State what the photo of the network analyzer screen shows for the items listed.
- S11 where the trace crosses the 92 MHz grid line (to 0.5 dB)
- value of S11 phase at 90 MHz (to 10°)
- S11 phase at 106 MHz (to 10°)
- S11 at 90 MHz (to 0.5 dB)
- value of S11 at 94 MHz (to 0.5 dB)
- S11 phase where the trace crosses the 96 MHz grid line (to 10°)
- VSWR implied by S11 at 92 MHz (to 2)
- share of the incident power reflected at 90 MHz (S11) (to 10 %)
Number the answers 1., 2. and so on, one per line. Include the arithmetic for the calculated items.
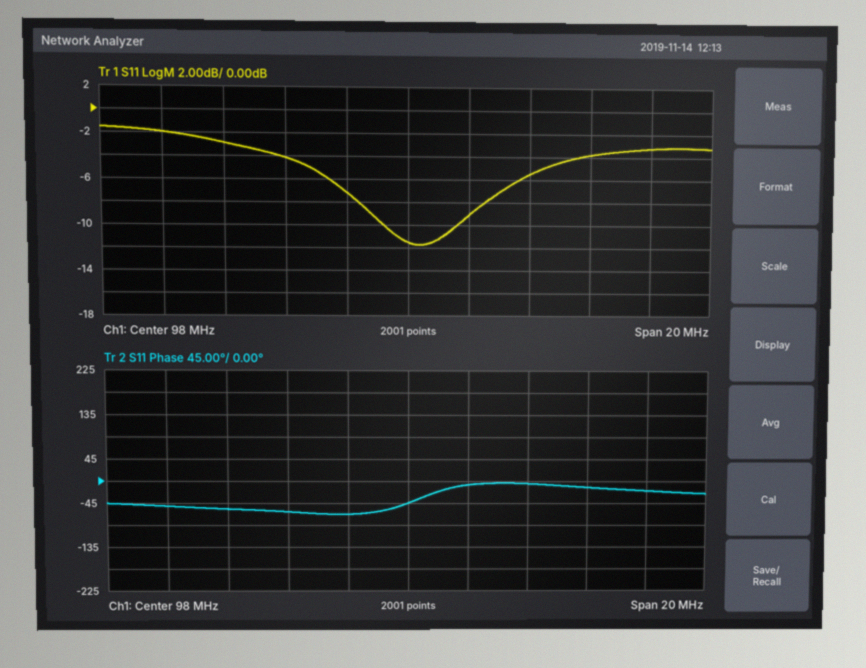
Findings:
1. -3.0 dB
2. -50°
3. -20°
4. -2.0 dB
5. -4.0 dB
6. -70°
7. |Γ| = 10^(-3/20) = 0.7079; VSWR = (1 + 0.7079)/(1 − 0.7079) ≈ 6
8. 10^(-2/10) ≈ 63.1 %, so 60 % to the nearest 10 %
